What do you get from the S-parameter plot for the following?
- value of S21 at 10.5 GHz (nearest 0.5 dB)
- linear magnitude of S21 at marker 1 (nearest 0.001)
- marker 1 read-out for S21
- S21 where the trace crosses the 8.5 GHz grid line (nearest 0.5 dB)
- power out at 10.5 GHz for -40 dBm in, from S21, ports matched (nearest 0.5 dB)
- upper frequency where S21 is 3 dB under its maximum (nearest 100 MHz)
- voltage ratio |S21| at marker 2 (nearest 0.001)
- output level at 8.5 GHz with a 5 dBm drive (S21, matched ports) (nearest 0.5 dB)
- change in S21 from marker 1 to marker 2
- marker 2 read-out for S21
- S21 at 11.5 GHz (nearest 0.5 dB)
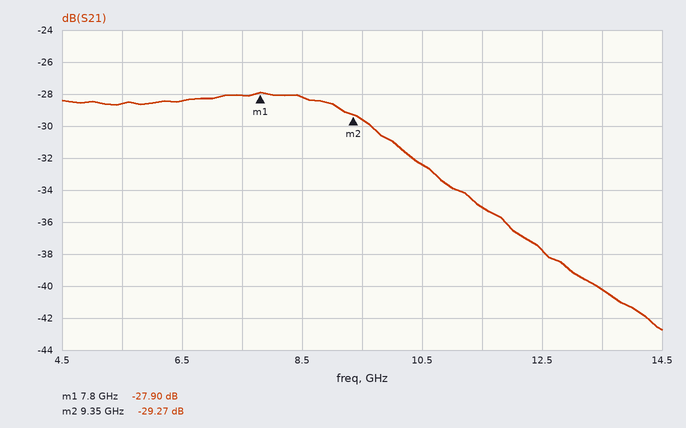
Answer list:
-32.5 dB
0.040
-27.90 dB
-28.0 dB
-72.5 dBm
10.0 GHz
0.034
-23.0 dBm
-1.37 dB
-29.27 dB
-35.0 dB
